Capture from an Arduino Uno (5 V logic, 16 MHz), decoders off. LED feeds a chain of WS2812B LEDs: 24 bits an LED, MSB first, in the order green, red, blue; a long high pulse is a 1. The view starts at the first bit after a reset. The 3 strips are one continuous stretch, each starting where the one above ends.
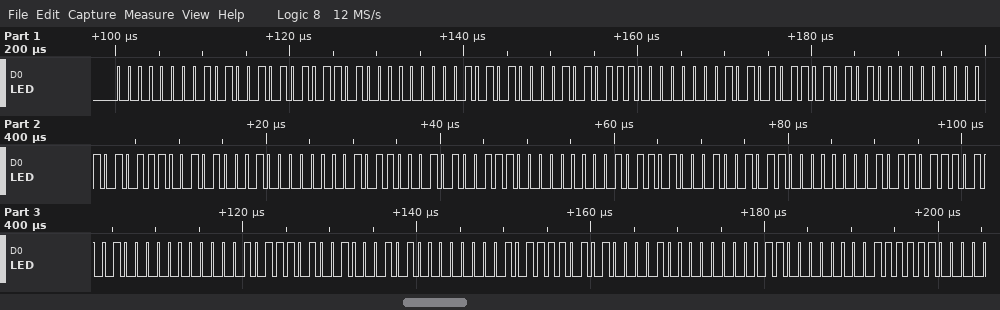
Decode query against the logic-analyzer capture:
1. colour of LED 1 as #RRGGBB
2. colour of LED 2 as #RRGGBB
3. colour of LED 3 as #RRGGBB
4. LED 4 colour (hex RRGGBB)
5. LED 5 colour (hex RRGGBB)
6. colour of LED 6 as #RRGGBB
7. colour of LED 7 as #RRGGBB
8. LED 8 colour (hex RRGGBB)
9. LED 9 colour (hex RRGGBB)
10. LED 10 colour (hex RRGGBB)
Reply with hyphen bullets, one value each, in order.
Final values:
- #A5005A
- #A80057
- #AB0054
- #AE0051
- #B1004E
- #B4004B
- #B70048
- #BA0045
- #BD0042
- #C0003F
